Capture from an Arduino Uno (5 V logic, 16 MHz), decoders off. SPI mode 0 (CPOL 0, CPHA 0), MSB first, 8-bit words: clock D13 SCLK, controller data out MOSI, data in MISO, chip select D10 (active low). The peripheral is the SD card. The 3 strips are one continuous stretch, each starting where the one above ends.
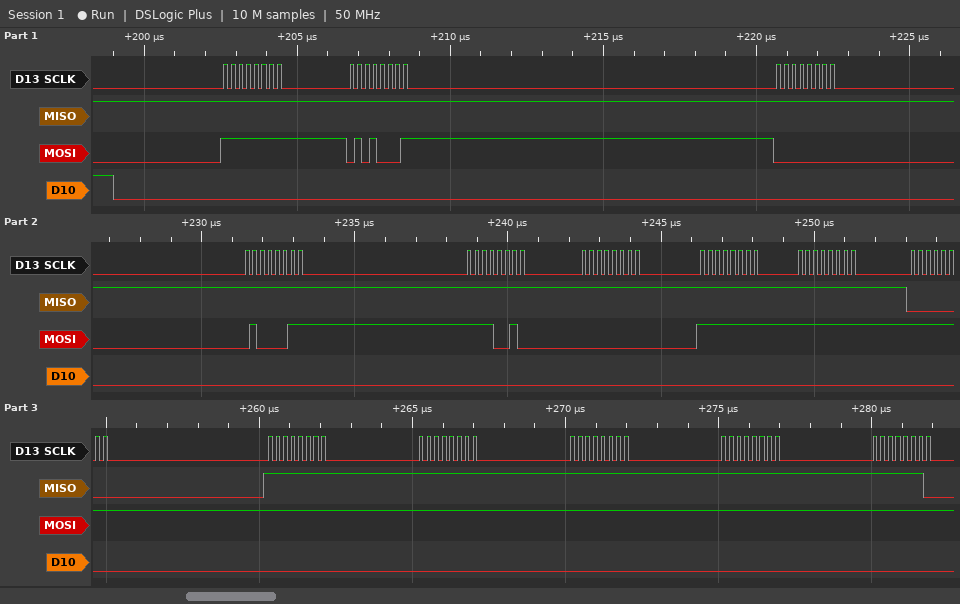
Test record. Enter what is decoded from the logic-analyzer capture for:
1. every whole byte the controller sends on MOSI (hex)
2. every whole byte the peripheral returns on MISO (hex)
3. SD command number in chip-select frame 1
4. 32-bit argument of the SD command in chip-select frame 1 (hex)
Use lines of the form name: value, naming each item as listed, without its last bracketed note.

every whole byte the controller sends on MOSI: FF 51 00 43 F2 00 FF FF FF FF FF FF FF FF
every whole byte the peripheral returns on MISO: FF FF FF FF FF FF FF FF 00 FF FF FF FF FE
SD command number in chip-select frame 1: CMD17
32-bit argument of the SD command in chip-select frame 1: 0x0043F200
